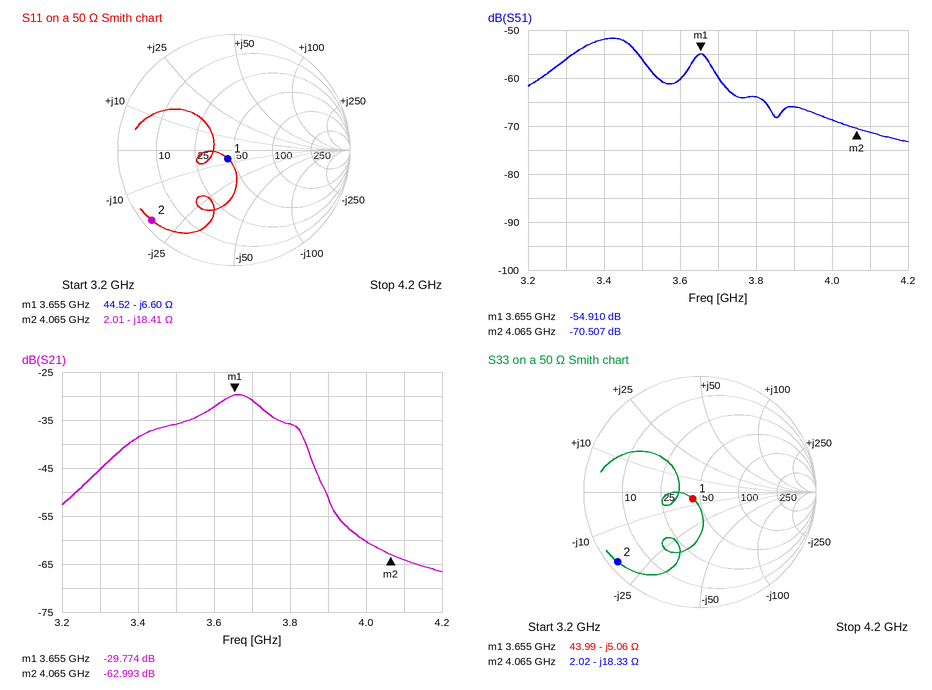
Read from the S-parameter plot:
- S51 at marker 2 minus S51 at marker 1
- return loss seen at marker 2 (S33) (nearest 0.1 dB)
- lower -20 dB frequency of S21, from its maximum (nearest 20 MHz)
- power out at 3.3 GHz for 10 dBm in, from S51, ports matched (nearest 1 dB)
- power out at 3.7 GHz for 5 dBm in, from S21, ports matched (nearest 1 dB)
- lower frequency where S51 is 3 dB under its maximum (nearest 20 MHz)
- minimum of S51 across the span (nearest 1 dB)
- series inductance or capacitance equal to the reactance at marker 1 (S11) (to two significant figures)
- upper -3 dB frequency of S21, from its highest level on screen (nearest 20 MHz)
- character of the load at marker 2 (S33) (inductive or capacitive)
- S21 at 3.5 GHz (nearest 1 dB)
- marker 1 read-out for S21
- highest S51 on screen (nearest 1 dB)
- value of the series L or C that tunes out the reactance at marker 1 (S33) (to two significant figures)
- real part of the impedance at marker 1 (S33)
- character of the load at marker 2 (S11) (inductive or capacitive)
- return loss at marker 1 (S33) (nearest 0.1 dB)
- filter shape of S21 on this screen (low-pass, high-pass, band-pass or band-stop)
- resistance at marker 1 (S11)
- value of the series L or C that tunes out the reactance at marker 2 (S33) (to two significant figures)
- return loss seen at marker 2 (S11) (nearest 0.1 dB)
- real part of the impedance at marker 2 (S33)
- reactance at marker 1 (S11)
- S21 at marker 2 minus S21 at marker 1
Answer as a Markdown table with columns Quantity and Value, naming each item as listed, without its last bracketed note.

| Quantity | Value |
|---|---|
| S51 at marker 2 minus S51 at marker 1 | -15.597 dB |
| return loss seen at marker 2 (S33) | 0.6 dB |
| lower -20 dB frequency of S21, from its maximum | 3.24 GHz |
| power out at 3.3 GHz for 10 dBm in, from S51, ports matched | -46 dBm |
| power out at 3.7 GHz for 5 dBm in, from S21, ports matched | -26 dBm |
| lower frequency where S51 is 3 dB under its maximum | 3.32 GHz |
| minimum of S51 across the span | -73 dB |
| series inductance or capacitance equal to the reactance at marker 1 (S11) | 6.6 pF |
| upper -3 dB frequency of S21, from its highest level on screen | 3.72 GHz |
| character of the load at marker 2 (S33) | capacitive |
| S21 at 3.5 GHz | -36 dB |
| marker 1 read-out for S21 | -29.774 dB |
| highest S51 on screen | -52 dB |
| value of the series L or C that tunes out the reactance at marker 1 (S33) | 220 pH |
| real part of the impedance at marker 1 | 43.99 Ω |
| character of the load at marker 2 (S11) | capacitive |
| return loss at marker 1 (S33) | 21.6 dB |
| filter shape of S21 on this screen | band-pass |
| resistance at marker 1 | 44.52 Ω |
| value of the series L or C that tunes out the reactance at marker 2 (S33) | 720 pH |
| return loss seen at marker 2 (S11) | 0.6 dB |
| real part of the impedance at marker 2 | 2.02 Ω |
| reactance at marker 1 | -6.60 Ω |
| S21 at marker 2 minus S21 at marker 1 | -33.219 dB |
